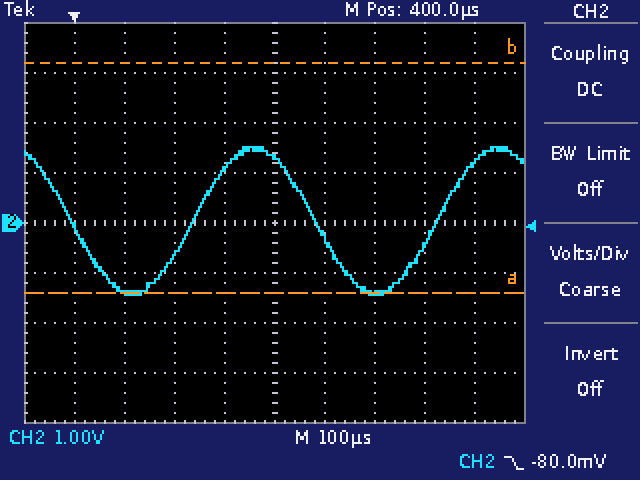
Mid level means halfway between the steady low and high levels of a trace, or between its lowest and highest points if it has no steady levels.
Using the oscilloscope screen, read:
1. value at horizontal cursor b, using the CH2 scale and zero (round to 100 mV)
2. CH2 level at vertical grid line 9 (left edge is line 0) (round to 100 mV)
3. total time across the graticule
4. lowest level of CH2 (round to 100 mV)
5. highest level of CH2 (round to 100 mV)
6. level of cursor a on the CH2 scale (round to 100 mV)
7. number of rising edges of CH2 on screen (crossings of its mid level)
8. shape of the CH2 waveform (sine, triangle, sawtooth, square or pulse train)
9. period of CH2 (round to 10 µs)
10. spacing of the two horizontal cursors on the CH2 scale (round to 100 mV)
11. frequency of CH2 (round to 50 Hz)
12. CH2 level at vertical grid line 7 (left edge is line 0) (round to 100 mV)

3.2 V
1.2 V
1 ms
-1.4 V
1.5 V
-1.4 V
2
sine
490 µs
4.6 V
2.05 kHz
-1.4 V
